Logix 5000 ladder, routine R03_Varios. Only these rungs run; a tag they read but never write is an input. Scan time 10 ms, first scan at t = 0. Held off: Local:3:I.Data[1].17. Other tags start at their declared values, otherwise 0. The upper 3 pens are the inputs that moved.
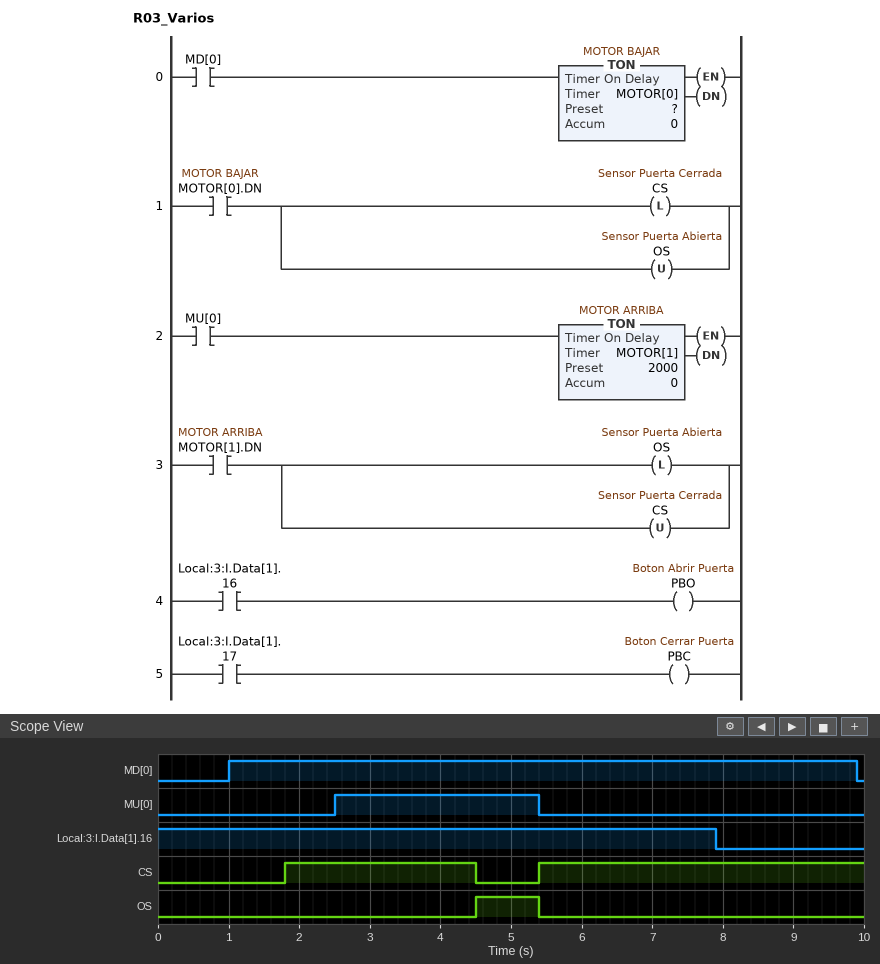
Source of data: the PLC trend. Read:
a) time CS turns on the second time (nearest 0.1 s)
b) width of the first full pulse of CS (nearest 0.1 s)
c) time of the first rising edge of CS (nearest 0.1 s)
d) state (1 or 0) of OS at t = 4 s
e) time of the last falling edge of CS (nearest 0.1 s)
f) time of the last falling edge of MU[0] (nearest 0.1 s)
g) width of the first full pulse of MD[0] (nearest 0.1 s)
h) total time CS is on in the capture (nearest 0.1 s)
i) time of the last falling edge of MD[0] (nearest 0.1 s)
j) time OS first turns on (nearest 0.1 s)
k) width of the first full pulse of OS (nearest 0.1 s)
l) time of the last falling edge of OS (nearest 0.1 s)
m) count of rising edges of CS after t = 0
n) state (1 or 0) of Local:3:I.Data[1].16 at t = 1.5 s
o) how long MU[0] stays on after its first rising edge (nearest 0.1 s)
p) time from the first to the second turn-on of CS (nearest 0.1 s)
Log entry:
5.4 s
2.7 s
1.8 s
0
4.5 s
5.4 s
8.9 s
7.3 s
9.9 s
4.5 s
0.9 s
5.4 s
2
1
2.9 s
3.6 s
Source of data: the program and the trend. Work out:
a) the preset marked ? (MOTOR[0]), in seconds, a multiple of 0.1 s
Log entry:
0.8 s
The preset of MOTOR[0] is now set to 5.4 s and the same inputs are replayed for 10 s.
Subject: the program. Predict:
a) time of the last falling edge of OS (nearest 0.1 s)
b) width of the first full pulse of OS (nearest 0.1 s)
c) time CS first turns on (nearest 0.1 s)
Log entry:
6.4 s
1.9 s
6.4 s
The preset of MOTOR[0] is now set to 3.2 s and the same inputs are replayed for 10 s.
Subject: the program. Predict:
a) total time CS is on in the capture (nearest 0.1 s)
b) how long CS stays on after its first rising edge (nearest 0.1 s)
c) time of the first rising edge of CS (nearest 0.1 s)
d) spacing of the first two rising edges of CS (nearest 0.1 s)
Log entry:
4.9 s
0.3 s
4.2 s
1.2 s
